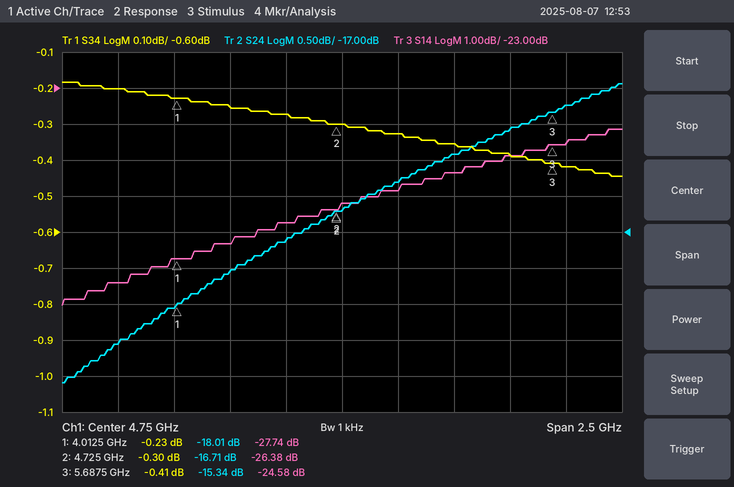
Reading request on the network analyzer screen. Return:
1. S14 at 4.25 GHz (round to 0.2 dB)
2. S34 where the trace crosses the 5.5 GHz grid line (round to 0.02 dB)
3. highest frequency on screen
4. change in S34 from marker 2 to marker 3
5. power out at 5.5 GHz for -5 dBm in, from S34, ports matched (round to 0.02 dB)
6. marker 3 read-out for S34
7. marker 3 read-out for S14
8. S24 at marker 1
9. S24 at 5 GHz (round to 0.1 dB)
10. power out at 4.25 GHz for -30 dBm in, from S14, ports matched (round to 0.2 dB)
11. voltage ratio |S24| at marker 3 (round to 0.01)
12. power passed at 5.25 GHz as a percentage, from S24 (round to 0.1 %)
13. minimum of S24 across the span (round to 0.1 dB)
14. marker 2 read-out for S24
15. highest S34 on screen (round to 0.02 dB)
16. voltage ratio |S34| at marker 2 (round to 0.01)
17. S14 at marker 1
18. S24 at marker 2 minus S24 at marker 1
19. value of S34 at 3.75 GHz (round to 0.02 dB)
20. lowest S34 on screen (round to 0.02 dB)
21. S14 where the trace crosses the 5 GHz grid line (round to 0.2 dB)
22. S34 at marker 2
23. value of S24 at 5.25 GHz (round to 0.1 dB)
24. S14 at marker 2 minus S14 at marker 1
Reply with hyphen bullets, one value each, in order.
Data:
- -27.4 dB
- -0.38 dB
- 6 GHz
- -0.11 dB
- -5.38 dBm
- -0.41 dB
- -24.58 dB
- -18.01 dB
- -16.3 dB
- -57.4 dBm
- 0.17
- 2.6 %
- -19.1 dB
- -16.71 dB
- -0.18 dB
- 0.97
- -27.74 dB
- 1.30 dB
- -0.20 dB
- -0.44 dB
- -25.8 dB
- -0.30 dB
- -15.9 dB
- 1.36 dB
